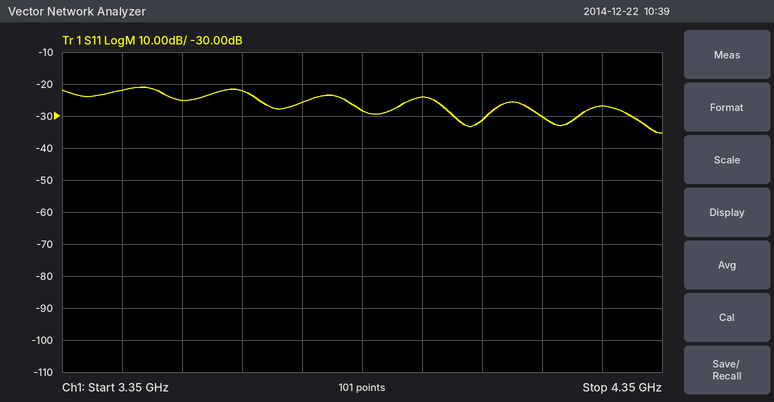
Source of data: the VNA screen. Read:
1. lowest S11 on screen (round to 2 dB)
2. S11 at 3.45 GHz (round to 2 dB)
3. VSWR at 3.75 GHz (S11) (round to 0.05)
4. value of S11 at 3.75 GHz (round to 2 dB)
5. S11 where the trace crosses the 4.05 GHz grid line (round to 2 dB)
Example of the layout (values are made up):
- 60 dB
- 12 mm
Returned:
- -36 dB
- -22 dB
- 1.10
- -26 dB
- -32 dB
